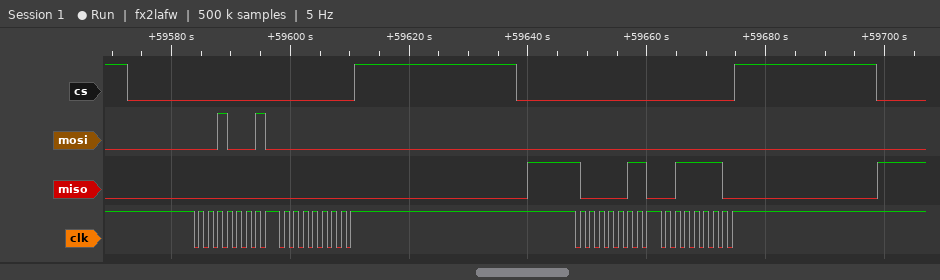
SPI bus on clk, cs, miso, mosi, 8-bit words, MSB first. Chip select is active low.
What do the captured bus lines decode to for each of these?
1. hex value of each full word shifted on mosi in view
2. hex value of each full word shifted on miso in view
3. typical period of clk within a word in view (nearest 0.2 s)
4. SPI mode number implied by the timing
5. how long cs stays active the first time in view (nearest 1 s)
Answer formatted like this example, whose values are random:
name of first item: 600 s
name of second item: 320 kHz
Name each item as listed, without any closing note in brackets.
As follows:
hex value of each full word shifted on mosi in view: 11, 00, 00, 00
hex value of each full word shifted on miso in view: 00, 00, 83, 3E
typical period of clk within a word in view: 1.6 s
SPI mode number implied by the timing: 2
how long cs stays active the first time in view: 38 s
